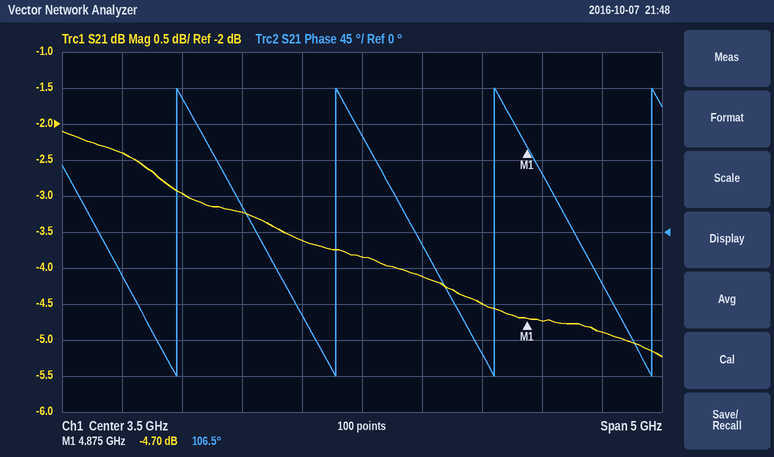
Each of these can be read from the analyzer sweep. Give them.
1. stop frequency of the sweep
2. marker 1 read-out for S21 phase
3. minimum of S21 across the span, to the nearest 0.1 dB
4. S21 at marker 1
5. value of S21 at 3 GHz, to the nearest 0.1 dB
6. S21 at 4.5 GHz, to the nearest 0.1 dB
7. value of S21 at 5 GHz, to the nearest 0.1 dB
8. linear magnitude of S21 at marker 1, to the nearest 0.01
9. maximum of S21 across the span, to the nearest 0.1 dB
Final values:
6 GHz
106.5°
-5.2 dB
-4.70 dB
-3.6 dB
-4.5 dB
-4.7 dB
0.58
-2.1 dB
